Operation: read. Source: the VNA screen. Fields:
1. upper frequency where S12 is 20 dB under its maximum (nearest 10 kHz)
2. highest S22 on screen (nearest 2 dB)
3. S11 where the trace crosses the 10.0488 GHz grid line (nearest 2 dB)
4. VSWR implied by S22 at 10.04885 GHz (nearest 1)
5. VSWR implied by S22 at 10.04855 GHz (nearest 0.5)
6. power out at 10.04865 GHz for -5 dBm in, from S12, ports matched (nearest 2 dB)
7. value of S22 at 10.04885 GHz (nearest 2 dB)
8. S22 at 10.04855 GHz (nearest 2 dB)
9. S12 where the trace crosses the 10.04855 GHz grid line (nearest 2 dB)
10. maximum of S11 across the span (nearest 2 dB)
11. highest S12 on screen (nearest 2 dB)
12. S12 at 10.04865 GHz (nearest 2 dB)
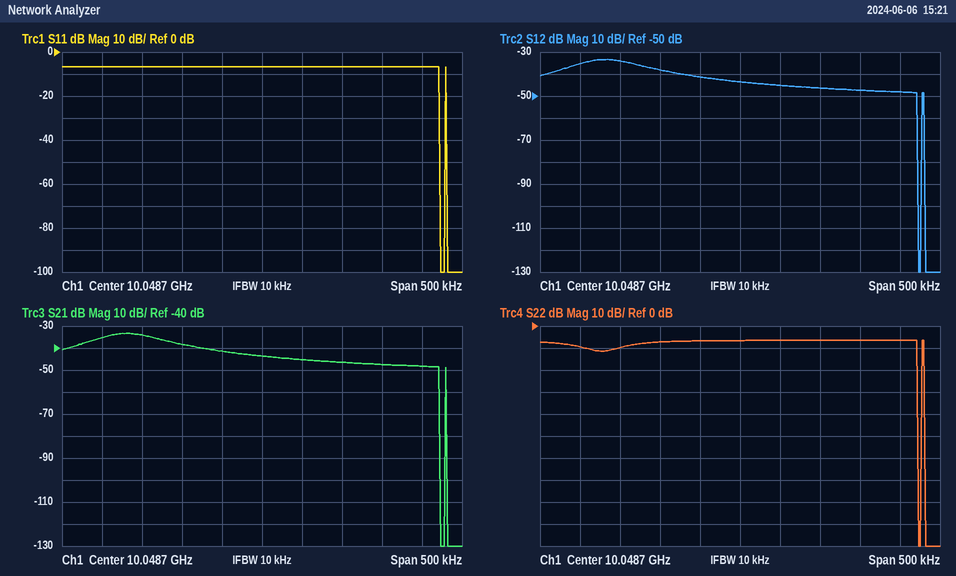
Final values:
10.04892 GHz
-6 dB
-6 dB
3
2.0
-46 dBm
-6 dB
-10 dB
-34 dB
-6 dB
-34 dB
-42 dB
